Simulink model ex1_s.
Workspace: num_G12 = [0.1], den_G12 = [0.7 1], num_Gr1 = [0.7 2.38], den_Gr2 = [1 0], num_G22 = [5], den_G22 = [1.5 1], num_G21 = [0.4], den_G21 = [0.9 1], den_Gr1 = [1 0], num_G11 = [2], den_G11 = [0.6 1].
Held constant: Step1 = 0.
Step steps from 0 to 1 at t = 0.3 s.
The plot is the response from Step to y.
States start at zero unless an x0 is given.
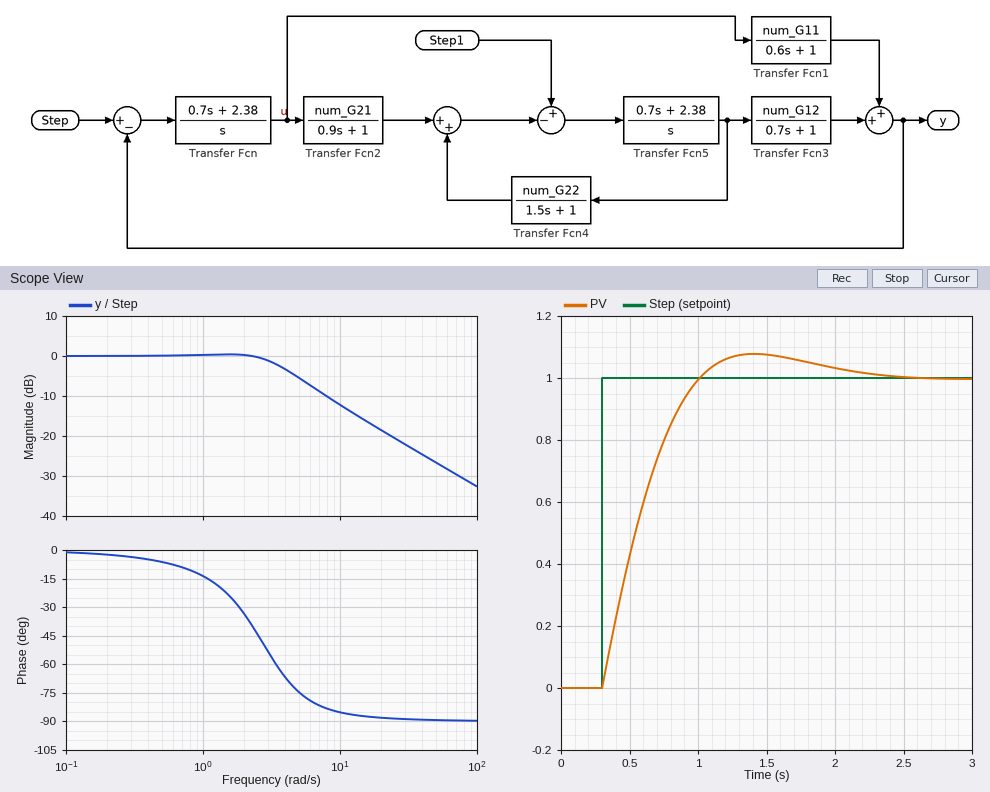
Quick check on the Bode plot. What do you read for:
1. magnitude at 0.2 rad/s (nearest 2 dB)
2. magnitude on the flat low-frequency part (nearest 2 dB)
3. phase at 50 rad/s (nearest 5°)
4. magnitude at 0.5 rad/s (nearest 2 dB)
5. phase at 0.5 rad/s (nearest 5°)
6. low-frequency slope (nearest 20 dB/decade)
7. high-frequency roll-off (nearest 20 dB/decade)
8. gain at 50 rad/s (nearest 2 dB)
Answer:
0 dB
0 dB
-90°
0 dB
-5°
0 dB/decade
-20 dB/decade
-26 dB
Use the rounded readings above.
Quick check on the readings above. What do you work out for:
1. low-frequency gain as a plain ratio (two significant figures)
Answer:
1.0
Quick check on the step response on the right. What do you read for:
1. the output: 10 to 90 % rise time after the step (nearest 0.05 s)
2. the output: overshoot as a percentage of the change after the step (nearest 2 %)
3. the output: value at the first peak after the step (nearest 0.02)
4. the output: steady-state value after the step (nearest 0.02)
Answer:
0.50 s
8 %
1.08
1.00
